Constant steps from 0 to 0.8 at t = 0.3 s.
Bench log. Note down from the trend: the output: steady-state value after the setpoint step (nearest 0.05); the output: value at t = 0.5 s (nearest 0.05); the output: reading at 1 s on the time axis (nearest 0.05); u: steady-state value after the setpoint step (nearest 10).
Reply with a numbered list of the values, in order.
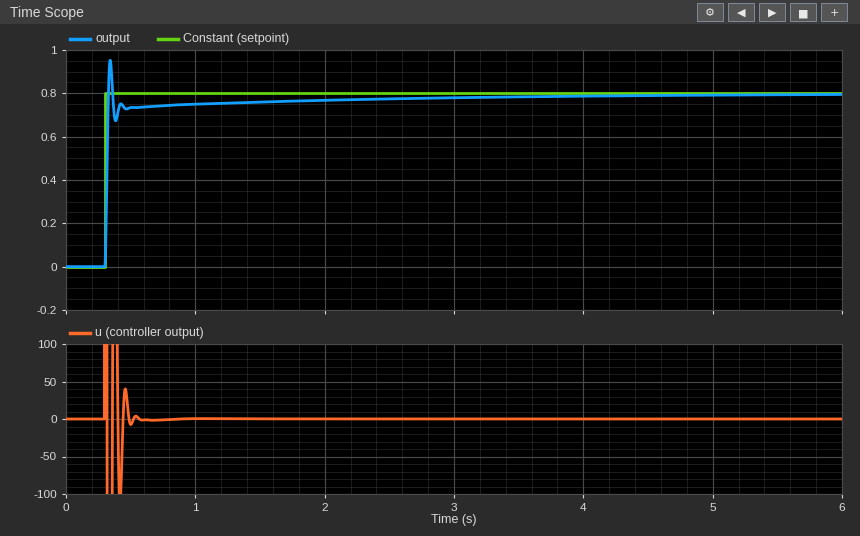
1. 0.80
2. 0.75
3. 0.75
4. 0
